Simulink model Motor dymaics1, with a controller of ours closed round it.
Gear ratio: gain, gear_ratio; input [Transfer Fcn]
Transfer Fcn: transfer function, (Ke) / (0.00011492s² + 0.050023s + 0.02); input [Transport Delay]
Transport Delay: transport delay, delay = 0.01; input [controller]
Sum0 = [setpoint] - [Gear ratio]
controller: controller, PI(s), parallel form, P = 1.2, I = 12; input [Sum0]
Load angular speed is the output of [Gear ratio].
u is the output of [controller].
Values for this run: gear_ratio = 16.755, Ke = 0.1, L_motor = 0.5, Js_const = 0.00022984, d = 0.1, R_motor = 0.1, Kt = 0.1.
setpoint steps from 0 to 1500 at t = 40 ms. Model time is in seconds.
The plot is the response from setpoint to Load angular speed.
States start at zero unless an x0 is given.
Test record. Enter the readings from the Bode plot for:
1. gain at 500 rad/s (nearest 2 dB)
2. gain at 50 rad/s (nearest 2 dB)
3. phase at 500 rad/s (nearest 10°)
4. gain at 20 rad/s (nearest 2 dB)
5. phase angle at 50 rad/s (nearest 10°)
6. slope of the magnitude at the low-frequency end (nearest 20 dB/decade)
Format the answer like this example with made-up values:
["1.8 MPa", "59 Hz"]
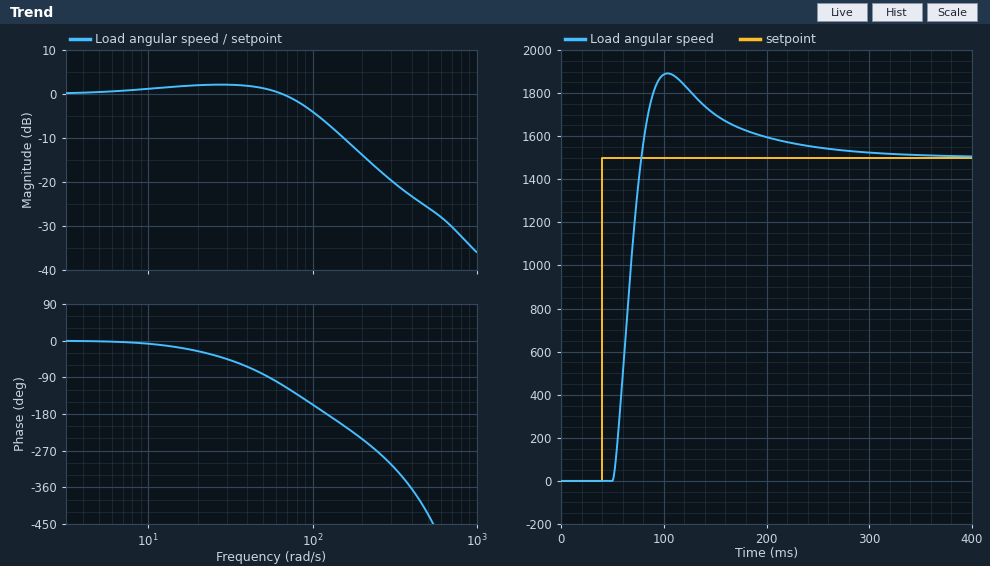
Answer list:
["-26 dB", "2 dB", "-420°", "2 dB", "-80°", "0 dB/decade"]
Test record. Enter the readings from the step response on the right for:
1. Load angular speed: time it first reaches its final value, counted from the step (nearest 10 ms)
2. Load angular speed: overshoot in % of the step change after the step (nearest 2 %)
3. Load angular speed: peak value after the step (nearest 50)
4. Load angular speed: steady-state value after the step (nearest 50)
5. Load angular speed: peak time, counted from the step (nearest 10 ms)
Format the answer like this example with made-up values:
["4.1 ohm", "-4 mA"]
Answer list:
["40 ms", "26 %", "1900", "1500", "60 ms"]
